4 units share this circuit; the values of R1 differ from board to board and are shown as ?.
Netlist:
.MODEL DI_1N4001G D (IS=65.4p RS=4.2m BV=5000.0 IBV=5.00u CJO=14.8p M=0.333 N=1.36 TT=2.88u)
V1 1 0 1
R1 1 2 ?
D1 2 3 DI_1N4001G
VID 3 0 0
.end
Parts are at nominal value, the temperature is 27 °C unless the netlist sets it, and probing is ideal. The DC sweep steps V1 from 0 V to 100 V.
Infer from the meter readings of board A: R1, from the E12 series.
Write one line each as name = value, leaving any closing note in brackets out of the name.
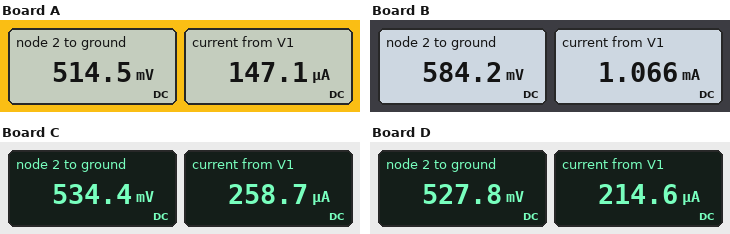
R1, from the E12 series = 3.3 kΩ
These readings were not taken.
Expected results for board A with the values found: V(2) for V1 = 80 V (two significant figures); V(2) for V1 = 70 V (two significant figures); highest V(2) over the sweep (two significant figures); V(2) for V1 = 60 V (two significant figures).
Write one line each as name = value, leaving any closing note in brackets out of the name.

V(2) for V1 = 80 V = 690 mV
V(2) for V1 = 70 V = 690 mV
highest V(2) over the sweep = 700 mV
V(2) for V1 = 60 V = 680 mV
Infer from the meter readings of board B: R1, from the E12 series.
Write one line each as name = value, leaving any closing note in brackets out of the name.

R1, from the E12 series = 390 Ω
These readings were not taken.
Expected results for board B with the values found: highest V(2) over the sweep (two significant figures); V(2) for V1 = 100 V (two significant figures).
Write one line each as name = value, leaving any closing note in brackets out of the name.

highest V(2) over the sweep = 780 mV
V(2) for V1 = 100 V = 780 mV
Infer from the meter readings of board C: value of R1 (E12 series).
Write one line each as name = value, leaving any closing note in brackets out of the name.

value of R1 = 1.8 kΩ
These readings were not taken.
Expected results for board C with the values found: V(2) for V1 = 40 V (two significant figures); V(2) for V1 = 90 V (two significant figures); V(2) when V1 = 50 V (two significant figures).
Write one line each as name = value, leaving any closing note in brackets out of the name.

V(2) for V1 = 40 V = 690 mV
V(2) for V1 = 90 V = 720 mV
V(2) when V1 = 50 V = 700 mV
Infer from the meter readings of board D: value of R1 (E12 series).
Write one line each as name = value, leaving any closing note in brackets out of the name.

value of R1 = 2.2 kΩ
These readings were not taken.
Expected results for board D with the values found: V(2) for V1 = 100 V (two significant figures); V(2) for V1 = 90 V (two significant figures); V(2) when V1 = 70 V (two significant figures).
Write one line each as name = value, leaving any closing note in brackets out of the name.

V(2) for V1 = 100 V = 720 mV
V(2) for V1 = 90 V = 710 mV
V(2) when V1 = 70 V = 700 mV
